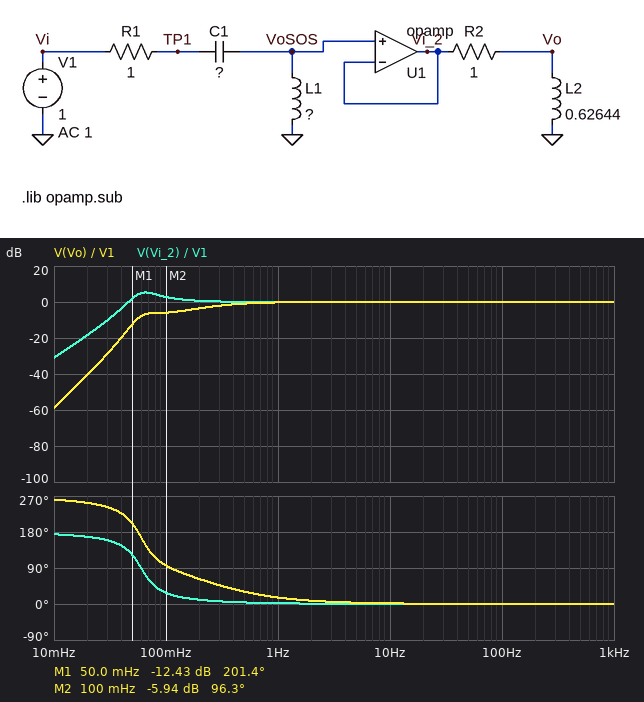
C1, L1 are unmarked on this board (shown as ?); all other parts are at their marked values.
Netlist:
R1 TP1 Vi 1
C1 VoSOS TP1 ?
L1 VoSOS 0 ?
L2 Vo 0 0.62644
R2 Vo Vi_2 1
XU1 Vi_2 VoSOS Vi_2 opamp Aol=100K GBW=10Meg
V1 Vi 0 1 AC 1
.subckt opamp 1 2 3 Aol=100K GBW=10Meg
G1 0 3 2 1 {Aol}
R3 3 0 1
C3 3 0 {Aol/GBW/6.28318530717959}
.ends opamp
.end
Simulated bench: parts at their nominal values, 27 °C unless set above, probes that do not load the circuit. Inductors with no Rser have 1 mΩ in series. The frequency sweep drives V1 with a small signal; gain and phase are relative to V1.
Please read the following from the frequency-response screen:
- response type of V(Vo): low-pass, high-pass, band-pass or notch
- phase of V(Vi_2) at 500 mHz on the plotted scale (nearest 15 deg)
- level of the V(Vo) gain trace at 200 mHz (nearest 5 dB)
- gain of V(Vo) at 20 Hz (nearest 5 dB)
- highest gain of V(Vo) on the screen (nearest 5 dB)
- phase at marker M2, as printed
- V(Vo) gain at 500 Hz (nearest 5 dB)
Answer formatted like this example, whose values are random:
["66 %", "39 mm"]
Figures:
["high-pass", "0 deg", "-5 dB", "0 dB", "0 dB", "96.3 deg", "0 dB"]
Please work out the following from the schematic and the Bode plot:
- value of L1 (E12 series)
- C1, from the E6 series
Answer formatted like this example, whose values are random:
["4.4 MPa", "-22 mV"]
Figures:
["4.7 H", "1.5 F"]
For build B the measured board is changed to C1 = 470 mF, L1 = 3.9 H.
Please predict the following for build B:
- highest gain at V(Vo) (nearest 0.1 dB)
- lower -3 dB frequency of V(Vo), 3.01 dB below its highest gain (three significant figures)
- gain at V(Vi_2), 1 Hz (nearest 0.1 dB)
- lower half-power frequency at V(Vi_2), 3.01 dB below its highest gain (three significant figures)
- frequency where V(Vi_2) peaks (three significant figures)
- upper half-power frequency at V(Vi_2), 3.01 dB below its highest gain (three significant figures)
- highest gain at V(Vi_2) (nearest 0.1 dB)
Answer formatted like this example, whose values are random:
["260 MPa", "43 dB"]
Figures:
["2.1 dB", "107 mHz", "0.1 dB", "104 mHz", "121 mHz", "152 mHz", "9.3 dB"]
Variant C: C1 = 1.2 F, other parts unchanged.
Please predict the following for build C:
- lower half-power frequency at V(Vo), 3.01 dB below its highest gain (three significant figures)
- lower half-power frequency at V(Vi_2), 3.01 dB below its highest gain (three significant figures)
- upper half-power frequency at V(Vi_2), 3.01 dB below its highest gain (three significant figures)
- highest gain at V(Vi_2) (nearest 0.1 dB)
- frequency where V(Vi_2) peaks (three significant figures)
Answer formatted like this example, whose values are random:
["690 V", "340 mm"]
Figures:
["217 mHz", "57.4 mHz", "108 mHz", "6.2 dB", "71.8 mHz"]
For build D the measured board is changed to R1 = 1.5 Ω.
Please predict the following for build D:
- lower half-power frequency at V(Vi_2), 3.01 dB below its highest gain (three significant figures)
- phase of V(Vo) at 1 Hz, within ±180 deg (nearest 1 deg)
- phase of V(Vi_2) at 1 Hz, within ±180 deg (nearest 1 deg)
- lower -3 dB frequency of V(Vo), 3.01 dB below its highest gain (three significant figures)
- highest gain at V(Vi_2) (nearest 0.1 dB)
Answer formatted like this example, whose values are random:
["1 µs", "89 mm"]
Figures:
["50.5 mHz", "17 deg", "3 deg", "235 mHz", "2.3 dB"]
